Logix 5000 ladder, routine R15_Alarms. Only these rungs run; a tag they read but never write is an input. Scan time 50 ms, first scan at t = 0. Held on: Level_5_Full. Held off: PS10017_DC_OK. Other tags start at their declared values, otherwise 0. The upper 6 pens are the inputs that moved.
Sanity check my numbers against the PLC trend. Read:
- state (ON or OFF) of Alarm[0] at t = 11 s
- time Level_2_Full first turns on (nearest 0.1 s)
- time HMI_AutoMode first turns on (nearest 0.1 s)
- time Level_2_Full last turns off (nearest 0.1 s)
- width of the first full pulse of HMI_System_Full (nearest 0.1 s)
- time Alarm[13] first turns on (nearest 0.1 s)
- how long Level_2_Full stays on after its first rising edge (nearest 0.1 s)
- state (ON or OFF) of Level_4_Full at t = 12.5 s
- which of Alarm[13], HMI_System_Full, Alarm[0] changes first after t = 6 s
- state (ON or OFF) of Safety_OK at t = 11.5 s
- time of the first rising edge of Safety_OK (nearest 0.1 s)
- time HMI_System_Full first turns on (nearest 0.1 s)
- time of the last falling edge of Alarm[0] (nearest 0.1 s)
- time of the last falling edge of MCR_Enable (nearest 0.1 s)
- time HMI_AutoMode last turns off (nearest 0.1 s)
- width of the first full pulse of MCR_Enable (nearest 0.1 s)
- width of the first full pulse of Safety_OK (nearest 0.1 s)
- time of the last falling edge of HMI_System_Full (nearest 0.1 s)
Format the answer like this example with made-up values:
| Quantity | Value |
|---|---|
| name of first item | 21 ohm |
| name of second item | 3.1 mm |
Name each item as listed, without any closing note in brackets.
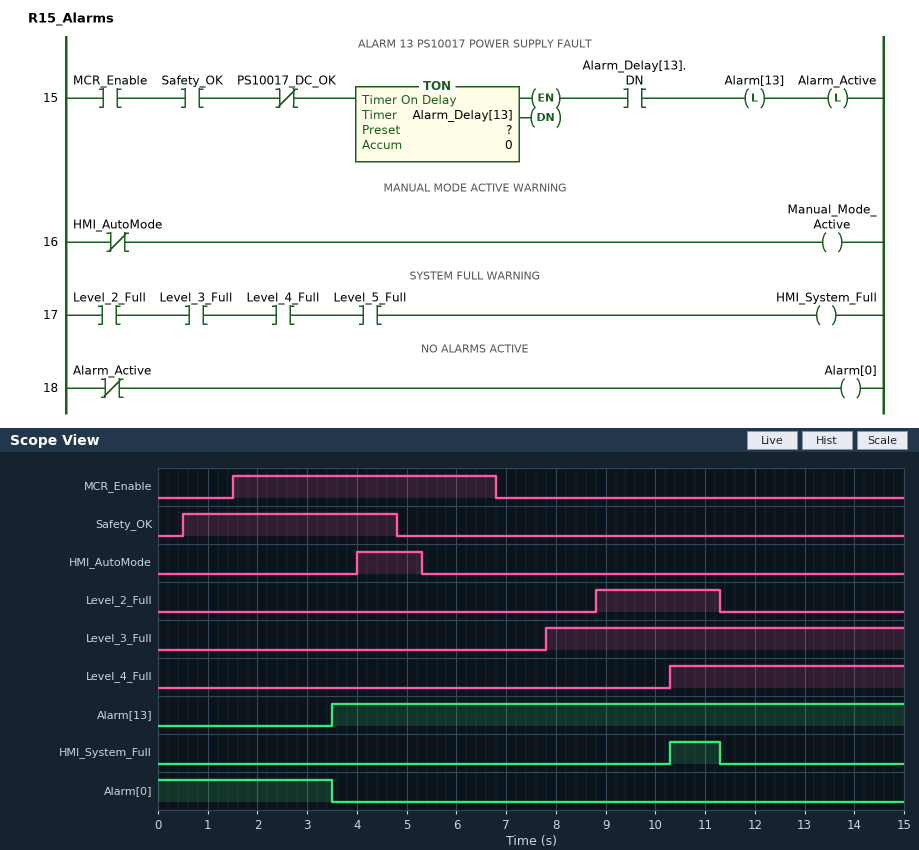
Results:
| Quantity | Value |
|---|---|
| state (ON or OFF) of Alarm[0] at t = 11 s | OFF |
| time Level_2_Full first turns on | 8.8 s |
| time HMI_AutoMode first turns on | 4.0 s |
| time Level_2_Full last turns off | 11.3 s |
| width of the first full pulse of HMI_System_Full | 1.0 s |
| time Alarm[13] first turns on | 3.5 s |
| how long Level_2_Full stays on after its first rising edge | 2.5 s |
| state (ON or OFF) of Level_4_Full at t = 12.5 s | ON |
| which of Alarm[13], HMI_System_Full, Alarm[0] changes first after t = 6 s | HMI_System_Full |
| state (ON or OFF) of Safety_OK at t = 11.5 s | OFF |
| time of the first rising edge of Safety_OK | 0.5 s |
| time HMI_System_Full first turns on | 10.3 s |
| time of the last falling edge of Alarm[0] | 3.5 s |
| time of the last falling edge of MCR_Enable | 6.8 s |
| time HMI_AutoMode last turns off | 5.3 s |
| width of the first full pulse of MCR_Enable | 5.3 s |
| width of the first full pulse of Safety_OK | 4.3 s |
| time of the last falling edge of HMI_System_Full | 11.3 s |
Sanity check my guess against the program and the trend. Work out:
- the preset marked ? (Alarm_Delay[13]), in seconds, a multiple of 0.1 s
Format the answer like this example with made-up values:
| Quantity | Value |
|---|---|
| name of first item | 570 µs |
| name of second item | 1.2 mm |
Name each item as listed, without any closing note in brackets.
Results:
| Quantity | Value |
|---|---|
| the preset marked ? (Alarm_Delay[13]), in seconds, a multiple of 0.1 s | 2.0 s |
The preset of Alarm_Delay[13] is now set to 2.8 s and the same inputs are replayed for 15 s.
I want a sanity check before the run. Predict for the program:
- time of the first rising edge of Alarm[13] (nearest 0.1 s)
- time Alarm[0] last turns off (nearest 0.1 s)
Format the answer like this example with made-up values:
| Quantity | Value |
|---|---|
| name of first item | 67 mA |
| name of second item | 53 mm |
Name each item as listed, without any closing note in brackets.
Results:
| Quantity | Value |
|---|---|
| time of the first rising edge of Alarm[13] | 4.3 s |
| time Alarm[0] last turns off | 4.3 s |
